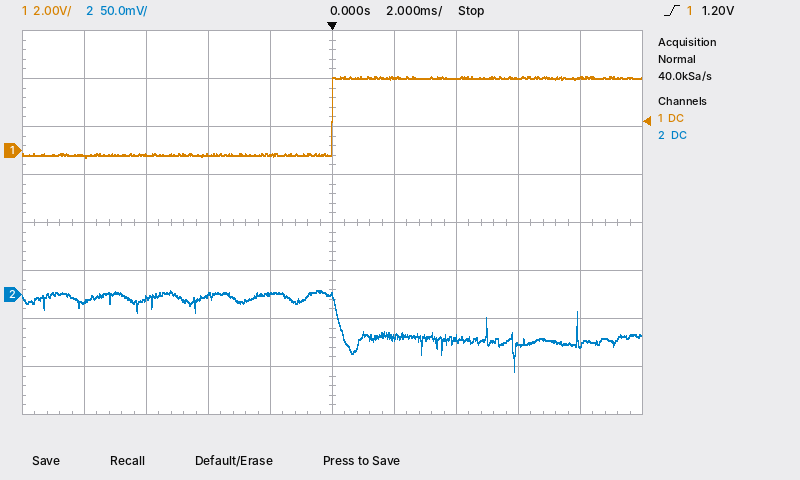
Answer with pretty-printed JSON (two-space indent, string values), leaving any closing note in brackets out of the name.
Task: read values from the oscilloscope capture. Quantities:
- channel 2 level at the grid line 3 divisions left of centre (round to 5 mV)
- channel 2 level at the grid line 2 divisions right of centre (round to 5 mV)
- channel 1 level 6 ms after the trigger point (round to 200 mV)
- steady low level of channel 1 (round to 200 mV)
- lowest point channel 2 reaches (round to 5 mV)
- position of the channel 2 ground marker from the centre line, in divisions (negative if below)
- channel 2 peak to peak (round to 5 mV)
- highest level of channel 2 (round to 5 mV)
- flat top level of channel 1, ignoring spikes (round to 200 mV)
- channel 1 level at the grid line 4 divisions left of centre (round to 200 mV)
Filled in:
{
  "channel 2 level at the grid line 3 divisions left of centre": "-5 mV",
  "channel 2 level at the grid line 2 divisions right of centre": "-45 mV",
  "channel 1 level 6 ms after the trigger point": "3.0 V",
  "steady low level of channel 1": "-200 mV",
  "lowest point channel 2 reaches": "-80 mV",
  "position of the channel 2 ground marker from the centre line, in divisions": "-1.5 div",
  "channel 2 peak to peak": "85 mV",
  "highest level of channel 2": "5 mV",
  "flat top level of channel 1, ignoring spikes": "3.0 V",
  "channel 1 level at the grid line 4 divisions left of centre": "-200 mV"
}
